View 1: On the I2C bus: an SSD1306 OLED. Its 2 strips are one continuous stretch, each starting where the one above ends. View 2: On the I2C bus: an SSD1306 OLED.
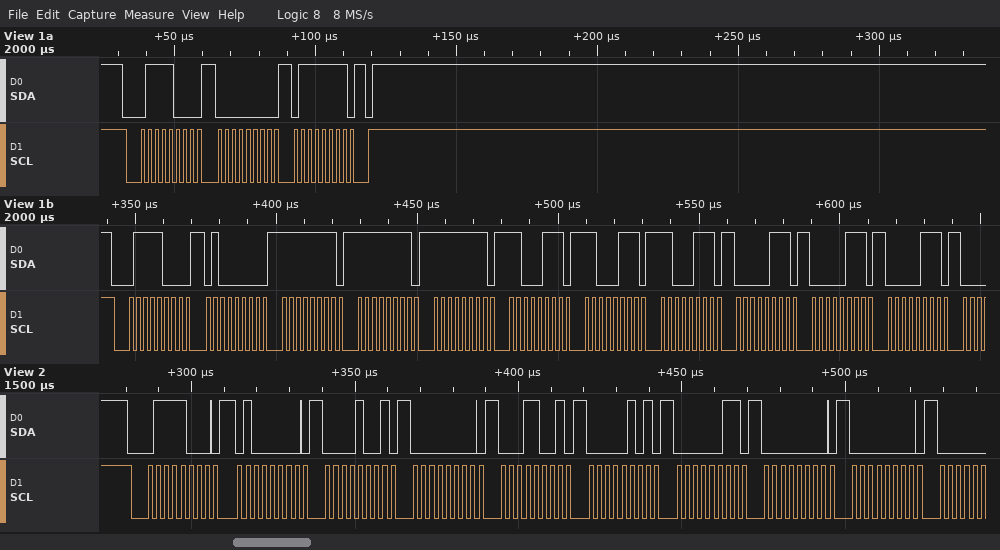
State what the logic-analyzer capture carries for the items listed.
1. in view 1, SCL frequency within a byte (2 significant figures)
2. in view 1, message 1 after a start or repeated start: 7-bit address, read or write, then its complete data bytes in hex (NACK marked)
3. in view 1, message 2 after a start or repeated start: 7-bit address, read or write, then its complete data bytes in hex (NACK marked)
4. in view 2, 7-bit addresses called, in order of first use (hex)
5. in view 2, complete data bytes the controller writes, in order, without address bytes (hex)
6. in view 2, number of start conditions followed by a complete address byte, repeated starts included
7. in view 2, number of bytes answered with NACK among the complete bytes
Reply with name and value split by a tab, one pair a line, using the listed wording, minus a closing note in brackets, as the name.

in view 1, SCL frequency within a byte	400 kHz
in view 1, message 1 after a start or repeated start: 7-bit address, read or write, then its complete data bytes in hex	0x3C write: 00 7F
in view 1, message 2 after a start or repeated start: 7-bit address, read or write, then its complete data bytes in hex	0x3C write: 40 FF FF FF C7 C7 C7 07 07 07
in view 2, 7-bit addresses called, in order of first use	0x3C
in view 2, complete data bytes the controller writes, in order, without address bytes	40 09 00 19 05 03 00 00
in view 2, number of start conditions followed by a complete address byte, repeated starts included	1
in view 2, number of bytes answered with NACK among the complete bytes	0
